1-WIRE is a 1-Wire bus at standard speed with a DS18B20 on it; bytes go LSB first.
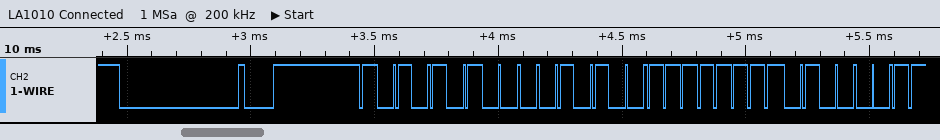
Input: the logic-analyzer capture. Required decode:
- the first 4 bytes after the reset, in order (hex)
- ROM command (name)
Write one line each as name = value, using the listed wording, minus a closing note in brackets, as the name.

the first 4 bytes after the reset, in order = 55 28 FF C2
ROM command = Match ROM
